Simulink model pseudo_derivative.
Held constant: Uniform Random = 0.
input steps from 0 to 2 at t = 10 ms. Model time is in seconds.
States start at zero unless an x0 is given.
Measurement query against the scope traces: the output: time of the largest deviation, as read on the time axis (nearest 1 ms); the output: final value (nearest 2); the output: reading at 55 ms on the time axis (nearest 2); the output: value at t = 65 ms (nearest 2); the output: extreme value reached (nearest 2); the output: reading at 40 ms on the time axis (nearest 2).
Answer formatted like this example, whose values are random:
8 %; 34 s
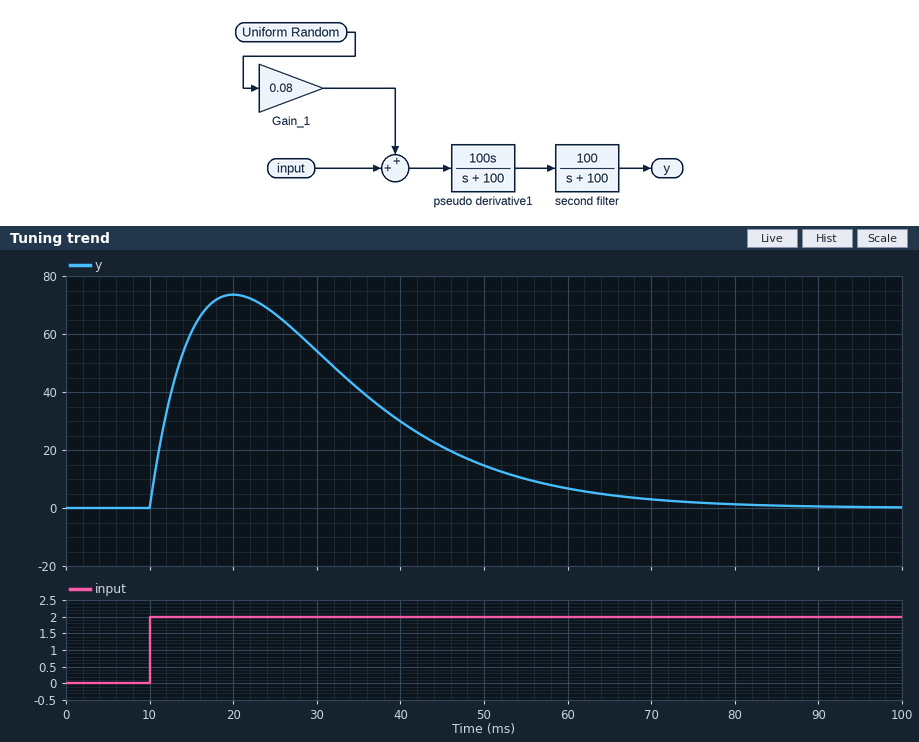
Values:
20 ms; 0; 10; 4; 74; 30
